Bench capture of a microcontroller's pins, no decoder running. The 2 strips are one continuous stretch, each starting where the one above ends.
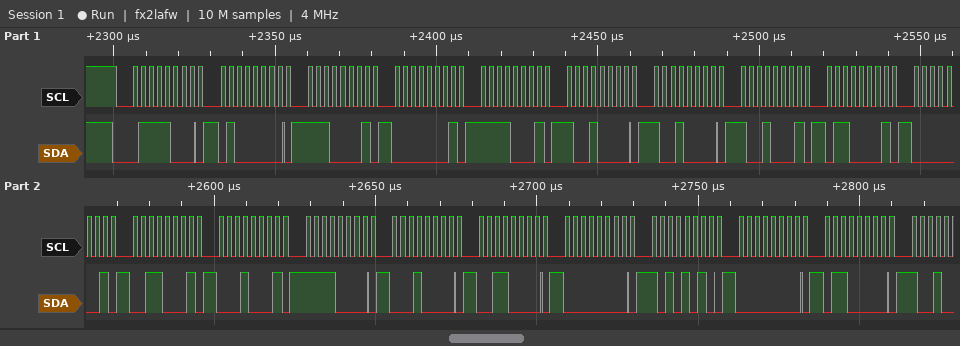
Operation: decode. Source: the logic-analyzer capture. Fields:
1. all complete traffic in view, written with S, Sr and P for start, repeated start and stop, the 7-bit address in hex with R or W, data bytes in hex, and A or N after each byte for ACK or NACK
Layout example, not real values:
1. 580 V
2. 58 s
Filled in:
1. S 3CW A 40 A E1 A 01 A F1 A 90 A 90 A 91 A 61 A 01 A 31 A 11 A F0 A 10 A 30 A 00 A AA A 00 A 60 A
